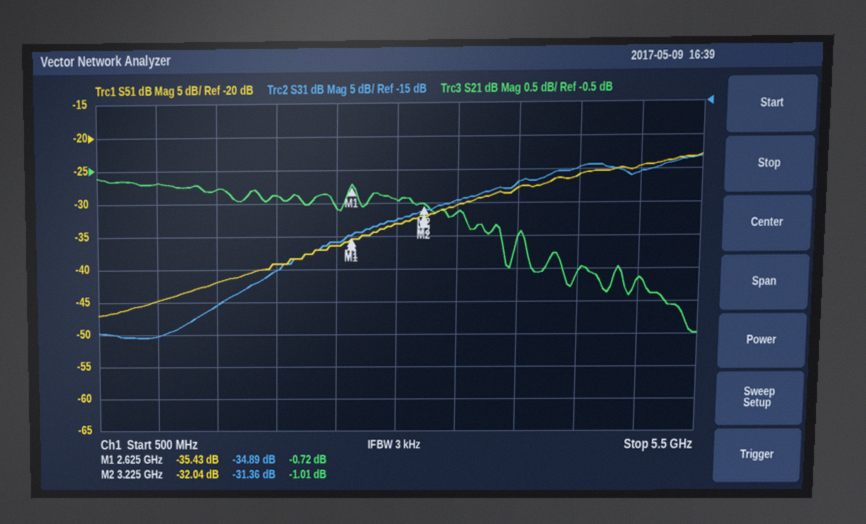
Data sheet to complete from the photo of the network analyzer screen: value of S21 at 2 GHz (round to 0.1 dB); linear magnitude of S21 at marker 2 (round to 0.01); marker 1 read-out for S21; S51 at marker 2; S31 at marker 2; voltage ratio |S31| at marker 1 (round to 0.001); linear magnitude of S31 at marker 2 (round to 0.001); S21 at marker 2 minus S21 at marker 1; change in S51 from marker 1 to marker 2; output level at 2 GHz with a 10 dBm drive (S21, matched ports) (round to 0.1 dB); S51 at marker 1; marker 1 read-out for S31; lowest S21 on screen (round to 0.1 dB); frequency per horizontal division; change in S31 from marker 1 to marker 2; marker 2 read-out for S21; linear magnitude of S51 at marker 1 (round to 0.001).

-0.9 dB
0.89
-0.72 dB
-32.04 dB
-31.36 dB
0.018
0.027
-0.29 dB
3.39 dB
9.1 dBm
-35.43 dB
-34.89 dB
-3.0 dB
500 MHz
3.53 dB
-1.01 dB
0.017
